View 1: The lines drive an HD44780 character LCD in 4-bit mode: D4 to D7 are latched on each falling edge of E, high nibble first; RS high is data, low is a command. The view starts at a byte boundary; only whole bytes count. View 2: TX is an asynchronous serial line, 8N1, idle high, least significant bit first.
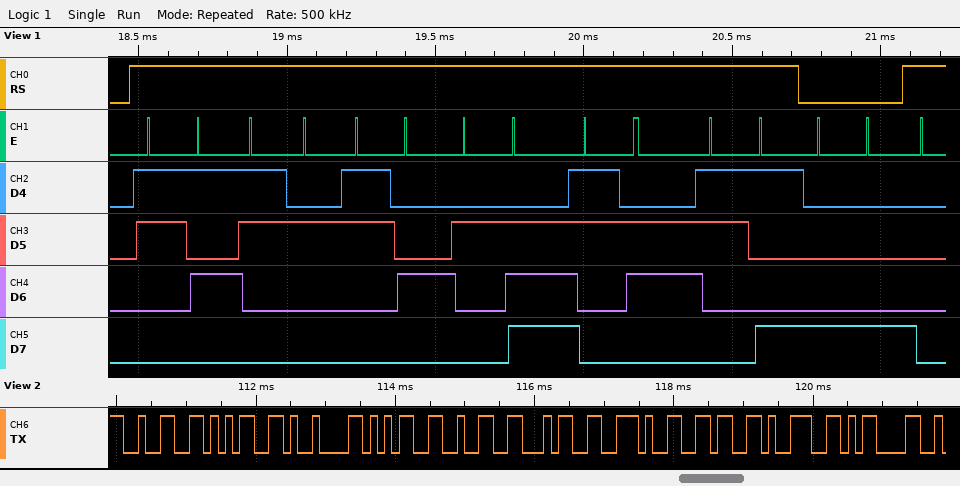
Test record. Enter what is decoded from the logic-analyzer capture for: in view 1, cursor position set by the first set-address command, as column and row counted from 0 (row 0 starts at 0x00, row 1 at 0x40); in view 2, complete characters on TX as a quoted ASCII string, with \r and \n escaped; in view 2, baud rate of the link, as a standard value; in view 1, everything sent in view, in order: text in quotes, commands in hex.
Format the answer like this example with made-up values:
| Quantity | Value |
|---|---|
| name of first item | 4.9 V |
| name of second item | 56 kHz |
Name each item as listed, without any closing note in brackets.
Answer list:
| Quantity | Value |
|---|---|
| in view 1, cursor position set by the first set-address command, as column and row counted from 0 | column 8, row 0 |
| in view 2, complete characters on TX as a quoted ASCII string, with \r and \n escaped | "25\t524.69\r" |
| in view 2, baud rate of the link, as a standard value | 9600 baud |
| in view 1, everything sent in view, in order: text in quotes, commands in hex | "524.69" 0x88 |
